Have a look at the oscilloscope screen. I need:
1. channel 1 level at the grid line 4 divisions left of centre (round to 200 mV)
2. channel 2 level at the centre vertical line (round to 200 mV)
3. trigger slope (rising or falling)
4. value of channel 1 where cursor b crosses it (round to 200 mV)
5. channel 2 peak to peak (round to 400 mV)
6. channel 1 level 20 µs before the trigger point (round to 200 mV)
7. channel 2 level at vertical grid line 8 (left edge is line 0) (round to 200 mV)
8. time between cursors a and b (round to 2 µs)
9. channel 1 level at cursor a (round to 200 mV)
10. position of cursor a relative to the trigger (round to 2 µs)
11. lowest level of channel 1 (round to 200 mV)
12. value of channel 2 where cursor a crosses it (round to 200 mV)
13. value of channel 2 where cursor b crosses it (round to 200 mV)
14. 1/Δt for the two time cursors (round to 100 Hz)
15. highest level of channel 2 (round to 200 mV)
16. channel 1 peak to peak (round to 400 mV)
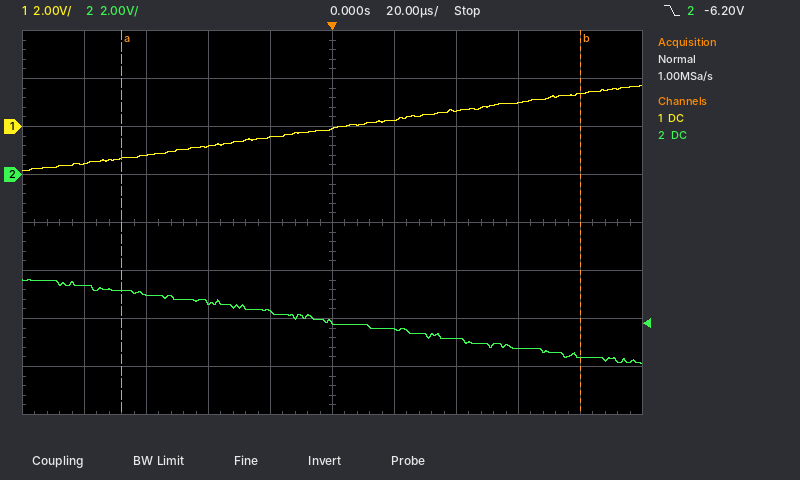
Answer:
-1.6 V
-6.2 V
falling
1.4 V
3.6 V
-400 mV
-7.2 V
148 µs
-1.4 V
-68 µs
-1.8 V
-4.8 V
-7.6 V
6.8 kHz
-4.4 V
3.6 V
